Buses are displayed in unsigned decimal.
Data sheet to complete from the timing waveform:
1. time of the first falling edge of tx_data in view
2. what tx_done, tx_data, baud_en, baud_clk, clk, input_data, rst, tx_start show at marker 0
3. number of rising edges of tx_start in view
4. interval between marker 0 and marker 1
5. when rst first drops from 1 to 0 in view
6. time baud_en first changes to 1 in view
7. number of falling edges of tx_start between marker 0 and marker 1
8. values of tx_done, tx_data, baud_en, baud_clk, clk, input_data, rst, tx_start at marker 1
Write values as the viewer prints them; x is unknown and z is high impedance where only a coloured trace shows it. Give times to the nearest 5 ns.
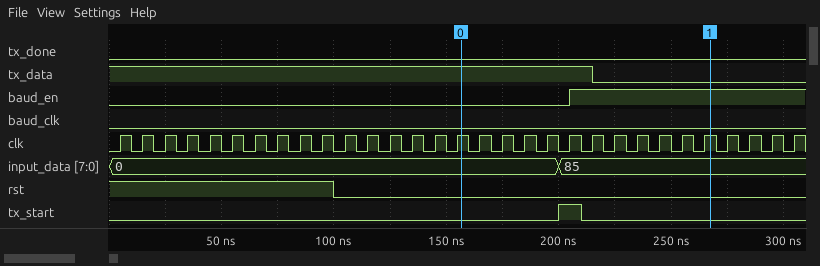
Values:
215 ns
tx_done=0, tx_data=1, baud_en=0, baud_clk=0, clk=1, input_data=0, rst=0, tx_start=0
1
110 ns
100 ns
205 ns
1
tx_done=0, tx_data=0, baud_en=1, baud_clk=0, clk=1, input_data=85, rst=0, tx_start=0
